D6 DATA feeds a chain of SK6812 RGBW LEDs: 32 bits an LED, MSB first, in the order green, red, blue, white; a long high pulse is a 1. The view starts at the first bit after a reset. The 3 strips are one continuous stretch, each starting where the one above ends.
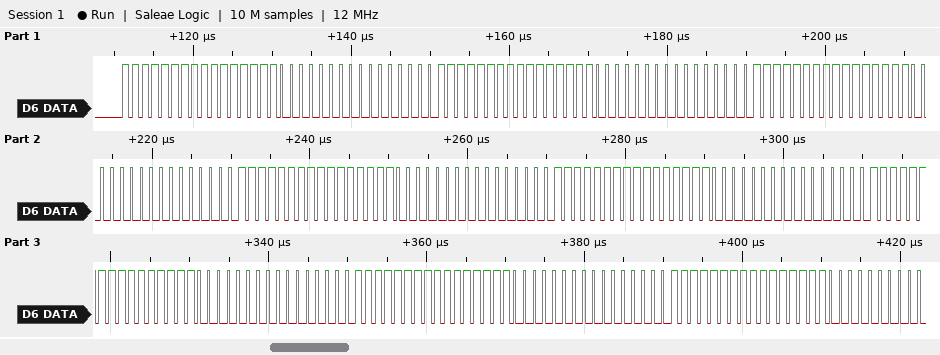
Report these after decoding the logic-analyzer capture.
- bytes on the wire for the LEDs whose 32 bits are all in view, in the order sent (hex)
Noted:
FF FF 00 00 FF FF 00 00 FF FF 00 00 FF FF 00 00 FF FF 00 00 FF FF 00 00 FF FF 00 00
